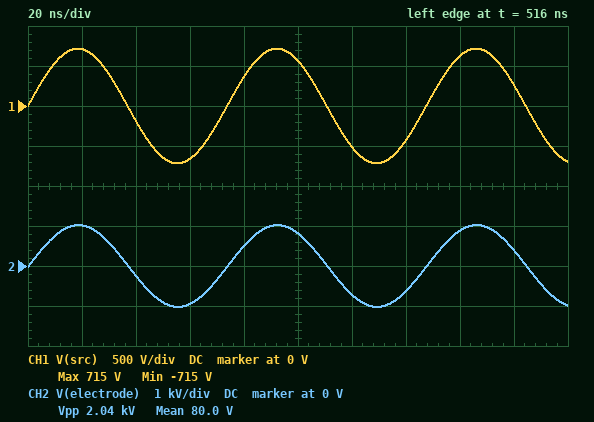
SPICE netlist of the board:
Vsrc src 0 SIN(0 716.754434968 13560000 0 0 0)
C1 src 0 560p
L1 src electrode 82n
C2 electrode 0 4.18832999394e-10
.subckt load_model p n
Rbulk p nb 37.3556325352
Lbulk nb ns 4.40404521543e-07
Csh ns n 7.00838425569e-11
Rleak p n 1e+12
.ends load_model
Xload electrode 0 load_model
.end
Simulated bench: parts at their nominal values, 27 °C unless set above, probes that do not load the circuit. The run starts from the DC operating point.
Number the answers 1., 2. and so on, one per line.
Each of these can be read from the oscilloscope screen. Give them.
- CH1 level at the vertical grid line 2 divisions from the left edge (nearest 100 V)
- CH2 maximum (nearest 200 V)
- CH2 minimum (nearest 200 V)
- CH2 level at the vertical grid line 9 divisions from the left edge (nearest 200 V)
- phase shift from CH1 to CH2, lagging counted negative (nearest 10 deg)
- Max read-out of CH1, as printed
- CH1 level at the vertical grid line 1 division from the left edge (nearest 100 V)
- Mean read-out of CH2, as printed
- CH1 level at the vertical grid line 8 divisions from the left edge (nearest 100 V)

1. -200 V
2. 1.0 kV
3. -1.0 kV
4. 400 V
5. 0 deg
6. 715 V
7. 700 V
8. 80.0 V
9. 600 V
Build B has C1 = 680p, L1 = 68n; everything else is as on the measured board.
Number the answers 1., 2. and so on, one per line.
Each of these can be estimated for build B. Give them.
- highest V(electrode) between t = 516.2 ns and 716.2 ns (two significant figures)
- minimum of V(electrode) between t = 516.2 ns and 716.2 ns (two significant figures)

1. 950 V
2. -950 V
